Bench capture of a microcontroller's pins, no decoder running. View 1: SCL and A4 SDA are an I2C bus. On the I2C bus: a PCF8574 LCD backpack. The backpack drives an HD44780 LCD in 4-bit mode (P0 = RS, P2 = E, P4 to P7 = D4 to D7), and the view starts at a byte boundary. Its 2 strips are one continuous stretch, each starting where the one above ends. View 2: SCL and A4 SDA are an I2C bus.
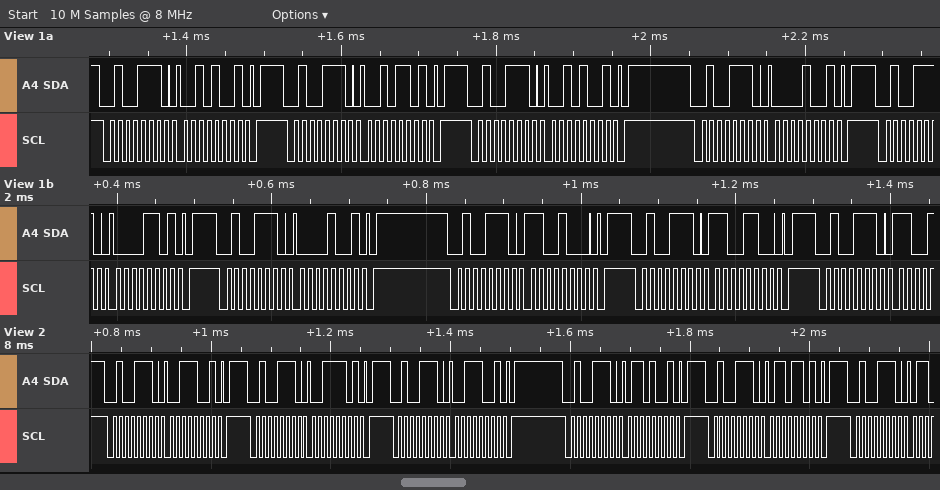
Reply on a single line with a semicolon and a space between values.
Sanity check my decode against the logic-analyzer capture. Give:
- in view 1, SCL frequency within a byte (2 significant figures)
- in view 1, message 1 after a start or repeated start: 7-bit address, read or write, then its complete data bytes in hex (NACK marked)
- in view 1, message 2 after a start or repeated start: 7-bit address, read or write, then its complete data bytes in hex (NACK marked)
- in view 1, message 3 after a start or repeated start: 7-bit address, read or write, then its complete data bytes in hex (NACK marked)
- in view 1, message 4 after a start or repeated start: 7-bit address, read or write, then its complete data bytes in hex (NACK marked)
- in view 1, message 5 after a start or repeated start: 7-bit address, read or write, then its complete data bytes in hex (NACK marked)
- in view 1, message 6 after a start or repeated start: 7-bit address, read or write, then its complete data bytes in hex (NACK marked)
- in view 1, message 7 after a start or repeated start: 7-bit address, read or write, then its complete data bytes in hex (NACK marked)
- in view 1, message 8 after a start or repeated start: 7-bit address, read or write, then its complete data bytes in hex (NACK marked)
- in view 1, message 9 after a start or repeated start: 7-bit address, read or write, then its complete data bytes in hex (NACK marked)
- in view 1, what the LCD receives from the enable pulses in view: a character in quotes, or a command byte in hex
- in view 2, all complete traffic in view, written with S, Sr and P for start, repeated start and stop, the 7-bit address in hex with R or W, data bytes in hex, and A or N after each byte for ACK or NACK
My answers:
100 kHz; 0x27 write: 29; 0x27 write: 2D; 0x27 write: 29; 0x27 write: 09; 0x27 write: 0D; 0x27 write: 09; 0x27 write: C8; 0x27 write: CC; 0x27 write; ' '; S 27W A 39 A P S 27W A 3D A P S 27W A 39 A P S 27W A 69 A P S 27W A 6D A P S 27W A
